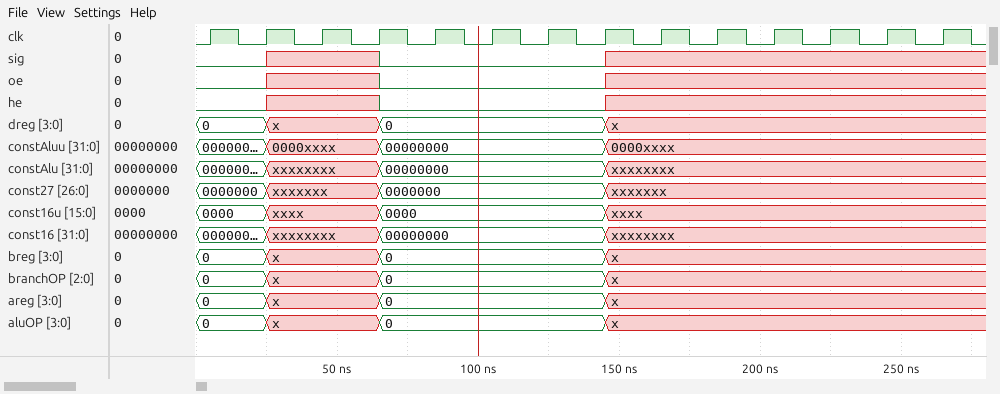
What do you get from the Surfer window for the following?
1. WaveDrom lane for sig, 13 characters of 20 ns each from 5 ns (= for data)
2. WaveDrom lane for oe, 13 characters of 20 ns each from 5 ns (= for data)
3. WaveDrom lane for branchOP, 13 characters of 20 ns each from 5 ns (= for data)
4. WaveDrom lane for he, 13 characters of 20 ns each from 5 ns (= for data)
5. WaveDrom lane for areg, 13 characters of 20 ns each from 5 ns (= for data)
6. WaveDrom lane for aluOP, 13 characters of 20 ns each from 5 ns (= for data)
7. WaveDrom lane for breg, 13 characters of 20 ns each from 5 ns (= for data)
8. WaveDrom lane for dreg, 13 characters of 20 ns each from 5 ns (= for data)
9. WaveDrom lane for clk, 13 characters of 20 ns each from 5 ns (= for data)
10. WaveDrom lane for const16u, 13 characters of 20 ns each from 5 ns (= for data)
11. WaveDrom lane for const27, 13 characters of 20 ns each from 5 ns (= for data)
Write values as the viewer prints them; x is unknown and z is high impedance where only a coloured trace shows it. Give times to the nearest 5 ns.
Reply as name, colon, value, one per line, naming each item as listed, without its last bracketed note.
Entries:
WaveDrom lane for sig, 13 characters of 20 ns each from 5 ns: {name: 'sig', wave: '0x.0...x.....'}
WaveDrom lane for oe, 13 characters of 20 ns each from 5 ns: {name: 'oe', wave: '0x.0...x.....'}
WaveDrom lane for branchOP, 13 characters of 20 ns each from 5 ns: {name: 'branchOP', wave: '=x.=...x.....', data: '0 0'}
WaveDrom lane for he, 13 characters of 20 ns each from 5 ns: {name: 'he', wave: '0x.0...x.....'}
WaveDrom lane for areg, 13 characters of 20 ns each from 5 ns: {name: 'areg', wave: '=x.=...x.....', data: '0 0'}
WaveDrom lane for aluOP, 13 characters of 20 ns each from 5 ns: {name: 'aluOP', wave: '=x.=...x.....', data: '0 0'}
WaveDrom lane for breg, 13 characters of 20 ns each from 5 ns: {name: 'breg', wave: '=x.=...x.....', data: '0 0'}
WaveDrom lane for dreg, 13 characters of 20 ns each from 5 ns: {name: 'dreg', wave: '=x.=...x.....', data: '0 0'}
WaveDrom lane for clk, 13 characters of 20 ns each from 5 ns: {name: 'clk', wave: 'p............'}
WaveDrom lane for const16u, 13 characters of 20 ns each from 5 ns: {name: 'const16u', wave: '=x.=...x.....', data: '0000 0000'}
WaveDrom lane for const27, 13 characters of 20 ns each from 5 ns: {name: 'const27', wave: '=x.=...x.....', data: '0000000 0000000'}
